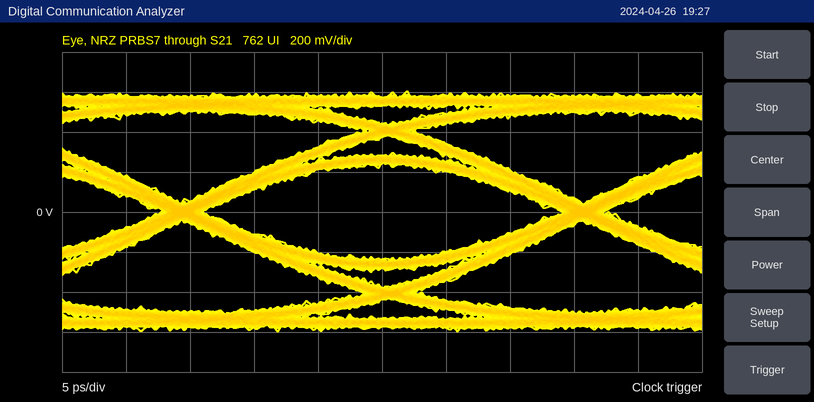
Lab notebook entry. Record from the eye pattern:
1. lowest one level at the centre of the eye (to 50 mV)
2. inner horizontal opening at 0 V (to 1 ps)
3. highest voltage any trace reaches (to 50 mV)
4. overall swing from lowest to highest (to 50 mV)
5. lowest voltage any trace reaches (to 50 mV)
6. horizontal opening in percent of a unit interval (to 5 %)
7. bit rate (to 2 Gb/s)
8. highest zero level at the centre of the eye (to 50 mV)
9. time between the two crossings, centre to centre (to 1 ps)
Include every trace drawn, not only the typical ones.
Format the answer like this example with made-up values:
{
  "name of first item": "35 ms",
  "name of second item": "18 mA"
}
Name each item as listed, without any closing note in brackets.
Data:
{
  "lowest one level at the centre of the eye": "250 mV",
  "inner horizontal opening at 0 V": "28 ps",
  "highest voltage any trace reaches": "600 mV",
  "overall swing from lowest to highest": "1.20 V",
  "lowest voltage any trace reaches": "-600 mV",
  "horizontal opening in percent of a unit interval": "90 %",
  "bit rate": "32 Gb/s",
  "highest zero level at the centre of the eye": "-250 mV",
  "time between the two crossings, centre to centre": "31 ps"
}
